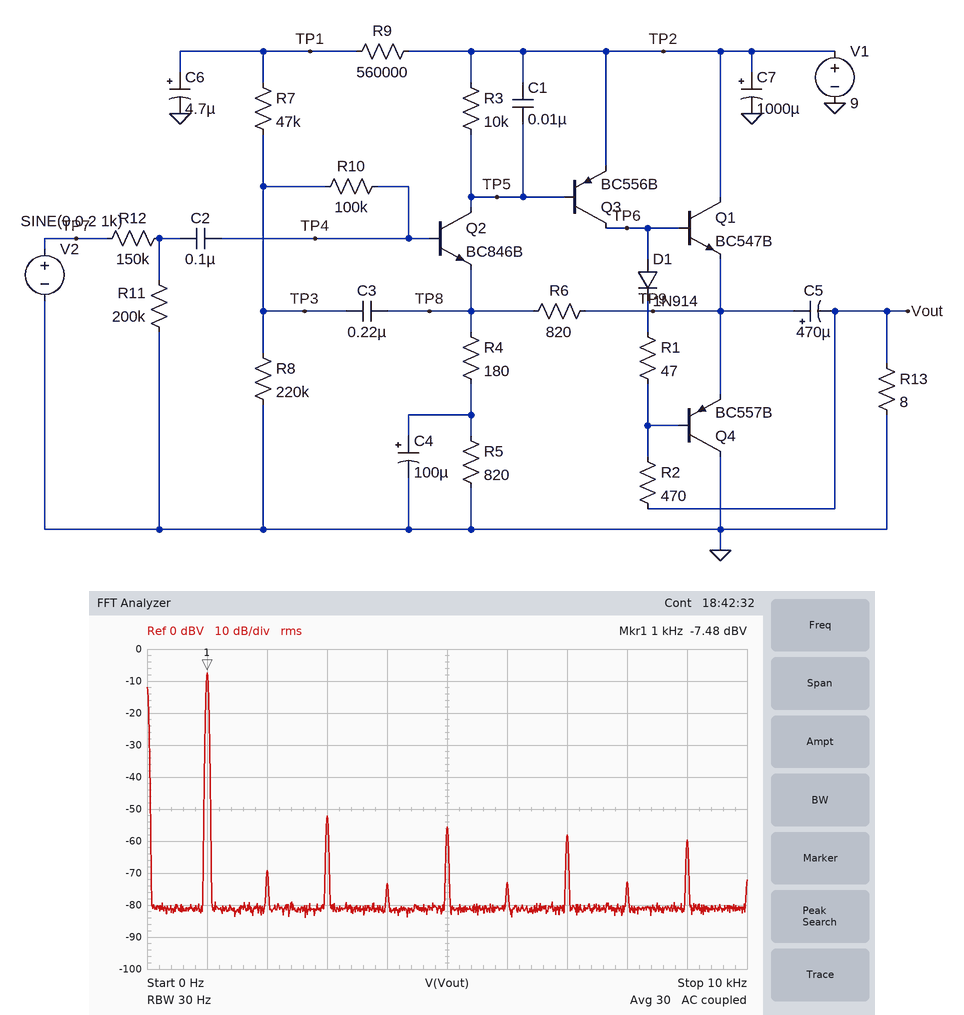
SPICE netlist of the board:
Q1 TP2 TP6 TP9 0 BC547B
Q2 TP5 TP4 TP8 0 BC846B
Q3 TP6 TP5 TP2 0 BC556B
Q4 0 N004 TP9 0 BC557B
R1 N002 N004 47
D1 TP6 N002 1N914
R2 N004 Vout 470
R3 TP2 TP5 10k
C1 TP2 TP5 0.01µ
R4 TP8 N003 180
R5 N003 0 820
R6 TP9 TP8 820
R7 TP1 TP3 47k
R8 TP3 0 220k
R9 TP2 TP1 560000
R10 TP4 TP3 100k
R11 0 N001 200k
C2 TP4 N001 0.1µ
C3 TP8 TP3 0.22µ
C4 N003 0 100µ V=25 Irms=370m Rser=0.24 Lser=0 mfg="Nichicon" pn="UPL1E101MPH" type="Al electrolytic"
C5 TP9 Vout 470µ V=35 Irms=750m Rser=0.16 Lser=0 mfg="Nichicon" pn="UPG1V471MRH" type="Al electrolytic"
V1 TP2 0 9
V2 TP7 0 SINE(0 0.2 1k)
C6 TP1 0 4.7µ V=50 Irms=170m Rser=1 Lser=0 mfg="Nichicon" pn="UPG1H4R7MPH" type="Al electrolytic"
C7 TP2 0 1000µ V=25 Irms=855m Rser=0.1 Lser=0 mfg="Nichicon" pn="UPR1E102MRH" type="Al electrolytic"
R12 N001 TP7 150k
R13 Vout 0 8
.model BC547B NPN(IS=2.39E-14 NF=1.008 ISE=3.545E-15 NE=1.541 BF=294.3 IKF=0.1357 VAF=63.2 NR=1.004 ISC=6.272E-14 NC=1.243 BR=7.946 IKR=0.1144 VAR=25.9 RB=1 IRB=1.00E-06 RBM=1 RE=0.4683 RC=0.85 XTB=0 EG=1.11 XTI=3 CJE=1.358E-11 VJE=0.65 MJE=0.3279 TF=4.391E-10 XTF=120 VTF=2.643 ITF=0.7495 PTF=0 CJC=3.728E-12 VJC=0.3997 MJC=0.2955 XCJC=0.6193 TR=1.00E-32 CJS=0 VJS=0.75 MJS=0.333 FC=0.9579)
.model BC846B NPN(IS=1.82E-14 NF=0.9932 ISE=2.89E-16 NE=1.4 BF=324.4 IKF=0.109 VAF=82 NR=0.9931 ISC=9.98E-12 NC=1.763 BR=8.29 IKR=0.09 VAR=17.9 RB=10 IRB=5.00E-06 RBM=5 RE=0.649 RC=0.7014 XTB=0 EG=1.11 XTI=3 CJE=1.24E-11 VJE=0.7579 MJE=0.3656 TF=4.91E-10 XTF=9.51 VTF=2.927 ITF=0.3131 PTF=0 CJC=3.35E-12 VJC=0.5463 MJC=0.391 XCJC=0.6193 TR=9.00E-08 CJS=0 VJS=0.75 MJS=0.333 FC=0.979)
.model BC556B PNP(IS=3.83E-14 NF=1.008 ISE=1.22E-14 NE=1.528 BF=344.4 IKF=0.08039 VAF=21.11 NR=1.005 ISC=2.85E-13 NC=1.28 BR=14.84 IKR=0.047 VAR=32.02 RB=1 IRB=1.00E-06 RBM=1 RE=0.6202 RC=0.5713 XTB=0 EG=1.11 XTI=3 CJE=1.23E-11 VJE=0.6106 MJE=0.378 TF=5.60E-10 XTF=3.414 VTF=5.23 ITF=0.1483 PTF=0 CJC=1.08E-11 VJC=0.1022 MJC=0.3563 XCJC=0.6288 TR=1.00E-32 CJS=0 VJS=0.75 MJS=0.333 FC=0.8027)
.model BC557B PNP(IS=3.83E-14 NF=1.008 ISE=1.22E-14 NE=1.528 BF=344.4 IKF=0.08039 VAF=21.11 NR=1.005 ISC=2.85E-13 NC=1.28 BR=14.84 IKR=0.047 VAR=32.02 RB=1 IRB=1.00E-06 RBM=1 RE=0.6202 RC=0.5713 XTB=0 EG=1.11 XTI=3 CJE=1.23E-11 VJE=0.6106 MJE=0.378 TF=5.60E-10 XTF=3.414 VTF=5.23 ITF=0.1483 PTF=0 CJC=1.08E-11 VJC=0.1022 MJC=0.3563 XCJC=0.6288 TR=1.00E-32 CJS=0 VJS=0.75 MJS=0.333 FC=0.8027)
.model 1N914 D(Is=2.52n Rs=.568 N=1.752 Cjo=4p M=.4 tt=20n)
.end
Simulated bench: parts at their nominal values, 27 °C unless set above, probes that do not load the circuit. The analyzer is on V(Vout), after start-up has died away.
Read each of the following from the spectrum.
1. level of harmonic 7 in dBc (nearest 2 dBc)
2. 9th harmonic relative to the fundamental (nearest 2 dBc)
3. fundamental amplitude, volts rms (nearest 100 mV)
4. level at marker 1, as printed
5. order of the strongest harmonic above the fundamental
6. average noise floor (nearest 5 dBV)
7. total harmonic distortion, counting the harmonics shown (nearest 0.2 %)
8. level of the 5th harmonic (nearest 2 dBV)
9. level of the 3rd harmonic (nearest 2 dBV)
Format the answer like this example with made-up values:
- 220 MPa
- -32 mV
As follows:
- -50 dBc
- -52 dBc
- 400 mV
- -7.48 dBV
- 3
- -80 dBV
- 0.8 %
- -56 dBV
- -52 dBV
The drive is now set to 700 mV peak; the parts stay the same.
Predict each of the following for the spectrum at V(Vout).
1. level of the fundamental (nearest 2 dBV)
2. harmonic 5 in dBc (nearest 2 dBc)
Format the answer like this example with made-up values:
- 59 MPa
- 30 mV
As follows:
- 4 dBV
- -56 dBc
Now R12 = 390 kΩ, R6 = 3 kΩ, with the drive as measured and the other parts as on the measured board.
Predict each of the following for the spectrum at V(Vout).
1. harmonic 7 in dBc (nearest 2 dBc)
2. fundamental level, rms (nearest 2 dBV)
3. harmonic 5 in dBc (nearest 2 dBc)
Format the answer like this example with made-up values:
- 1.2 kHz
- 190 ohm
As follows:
- -58 dBc
- -2 dBV
- -54 dBc
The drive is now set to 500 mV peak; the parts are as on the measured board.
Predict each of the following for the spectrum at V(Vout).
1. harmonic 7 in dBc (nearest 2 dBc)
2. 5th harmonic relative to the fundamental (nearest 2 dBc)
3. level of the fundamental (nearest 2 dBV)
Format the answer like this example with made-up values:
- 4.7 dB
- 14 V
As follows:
- -58 dBc
- -56 dBc
- 0 dBV
